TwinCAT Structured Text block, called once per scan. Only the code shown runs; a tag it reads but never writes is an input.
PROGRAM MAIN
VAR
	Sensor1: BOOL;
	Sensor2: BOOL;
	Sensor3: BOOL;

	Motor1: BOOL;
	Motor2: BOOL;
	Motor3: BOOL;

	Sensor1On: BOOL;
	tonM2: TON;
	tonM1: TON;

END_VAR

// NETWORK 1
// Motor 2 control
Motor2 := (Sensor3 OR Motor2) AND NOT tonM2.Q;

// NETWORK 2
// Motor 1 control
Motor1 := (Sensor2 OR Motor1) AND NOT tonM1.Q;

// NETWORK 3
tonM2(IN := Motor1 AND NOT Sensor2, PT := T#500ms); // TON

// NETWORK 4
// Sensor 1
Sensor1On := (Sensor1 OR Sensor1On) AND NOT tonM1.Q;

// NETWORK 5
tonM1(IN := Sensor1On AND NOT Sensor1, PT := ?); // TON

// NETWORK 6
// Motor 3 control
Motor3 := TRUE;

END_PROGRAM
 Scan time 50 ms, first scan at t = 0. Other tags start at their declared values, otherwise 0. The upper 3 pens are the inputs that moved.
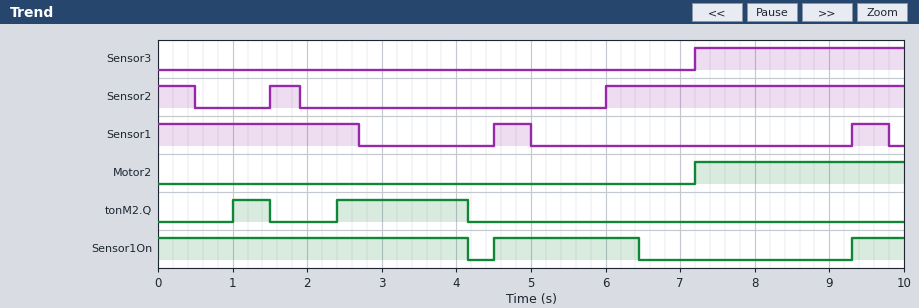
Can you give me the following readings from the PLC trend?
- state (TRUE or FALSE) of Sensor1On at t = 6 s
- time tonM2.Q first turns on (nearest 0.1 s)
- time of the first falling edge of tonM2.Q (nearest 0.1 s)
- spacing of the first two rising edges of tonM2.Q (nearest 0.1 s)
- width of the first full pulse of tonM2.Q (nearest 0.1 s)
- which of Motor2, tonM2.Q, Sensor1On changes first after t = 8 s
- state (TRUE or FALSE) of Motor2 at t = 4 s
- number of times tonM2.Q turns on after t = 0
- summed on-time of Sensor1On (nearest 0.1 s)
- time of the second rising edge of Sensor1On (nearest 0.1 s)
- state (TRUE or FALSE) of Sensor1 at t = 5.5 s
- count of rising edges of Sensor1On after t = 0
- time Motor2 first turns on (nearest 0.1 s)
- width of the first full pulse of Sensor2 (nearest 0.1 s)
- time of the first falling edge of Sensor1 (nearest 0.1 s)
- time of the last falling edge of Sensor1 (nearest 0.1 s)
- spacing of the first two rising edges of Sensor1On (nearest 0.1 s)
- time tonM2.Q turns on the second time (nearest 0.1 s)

TRUE
1.0 s
1.5 s
1.4 s
0.5 s
Sensor1On
FALSE
2
6.8 s
9.3 s
FALSE
2
7.2 s
0.4 s
2.7 s
9.8 s
4.8 s
2.4 s
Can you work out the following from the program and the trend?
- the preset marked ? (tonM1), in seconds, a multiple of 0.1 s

1.4 s
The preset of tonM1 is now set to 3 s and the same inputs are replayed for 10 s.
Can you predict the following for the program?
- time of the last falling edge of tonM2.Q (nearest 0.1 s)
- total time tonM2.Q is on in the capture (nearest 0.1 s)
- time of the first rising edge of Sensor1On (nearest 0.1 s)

6.0 s
4.1 s
9.3 s
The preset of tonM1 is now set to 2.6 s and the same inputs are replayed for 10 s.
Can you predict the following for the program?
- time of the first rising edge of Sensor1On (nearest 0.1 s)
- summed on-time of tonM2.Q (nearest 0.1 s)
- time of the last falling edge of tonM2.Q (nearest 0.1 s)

9.3 s
4.1 s
6.0 s
